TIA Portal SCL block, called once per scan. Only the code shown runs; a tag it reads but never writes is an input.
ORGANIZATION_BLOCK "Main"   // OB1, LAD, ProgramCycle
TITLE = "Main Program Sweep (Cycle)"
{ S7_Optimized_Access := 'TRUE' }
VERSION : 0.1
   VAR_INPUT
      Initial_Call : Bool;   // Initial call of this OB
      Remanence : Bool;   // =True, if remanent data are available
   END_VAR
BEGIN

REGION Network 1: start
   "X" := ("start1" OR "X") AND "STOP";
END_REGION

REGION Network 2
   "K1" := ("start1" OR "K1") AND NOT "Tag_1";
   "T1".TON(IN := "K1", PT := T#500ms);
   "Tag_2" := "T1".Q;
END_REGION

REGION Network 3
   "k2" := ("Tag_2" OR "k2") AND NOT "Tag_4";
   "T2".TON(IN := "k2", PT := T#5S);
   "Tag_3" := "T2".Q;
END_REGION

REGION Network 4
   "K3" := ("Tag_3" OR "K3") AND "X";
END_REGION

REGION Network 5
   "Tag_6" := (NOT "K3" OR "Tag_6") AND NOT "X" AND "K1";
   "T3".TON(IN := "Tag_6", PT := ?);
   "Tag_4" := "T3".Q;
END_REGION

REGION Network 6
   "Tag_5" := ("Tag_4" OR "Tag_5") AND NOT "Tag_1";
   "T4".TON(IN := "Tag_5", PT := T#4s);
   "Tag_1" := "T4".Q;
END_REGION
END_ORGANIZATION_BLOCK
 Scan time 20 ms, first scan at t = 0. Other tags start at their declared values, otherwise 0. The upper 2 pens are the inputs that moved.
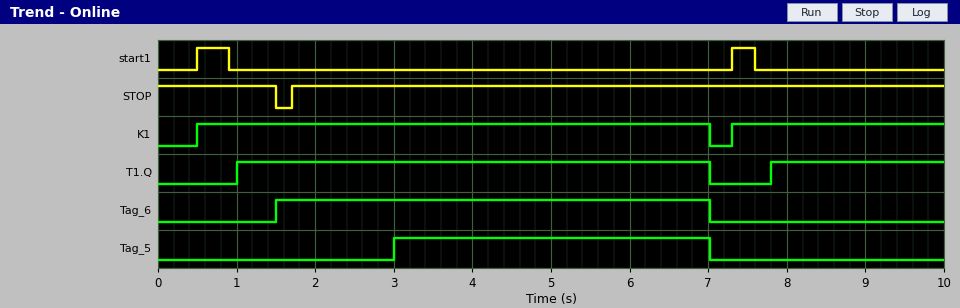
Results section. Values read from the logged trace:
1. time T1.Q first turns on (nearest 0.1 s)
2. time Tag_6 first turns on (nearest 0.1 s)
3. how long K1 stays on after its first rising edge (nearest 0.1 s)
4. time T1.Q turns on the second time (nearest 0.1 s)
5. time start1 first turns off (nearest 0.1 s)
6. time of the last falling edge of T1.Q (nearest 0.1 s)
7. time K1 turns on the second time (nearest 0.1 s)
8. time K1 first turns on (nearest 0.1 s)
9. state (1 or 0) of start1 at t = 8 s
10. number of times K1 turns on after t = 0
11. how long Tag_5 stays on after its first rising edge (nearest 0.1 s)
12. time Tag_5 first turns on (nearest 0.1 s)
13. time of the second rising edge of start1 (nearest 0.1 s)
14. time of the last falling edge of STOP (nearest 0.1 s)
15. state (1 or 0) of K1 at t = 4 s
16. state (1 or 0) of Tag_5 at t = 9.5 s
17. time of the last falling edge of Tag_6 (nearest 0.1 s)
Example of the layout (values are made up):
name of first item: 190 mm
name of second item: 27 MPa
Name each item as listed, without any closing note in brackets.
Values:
time T1.Q first turns on: 1.0 s
time Tag_6 first turns on: 1.5 s
how long K1 stays on after its first rising edge: 6.5 s
time T1.Q turns on the second time: 7.8 s
time start1 first turns off: 0.9 s
time of the last falling edge of T1.Q: 7.0 s
time K1 turns on the second time: 7.3 s
time K1 first turns on: 0.5 s
state (1 or 0) of start1 at t = 8 s: 0
number of times K1 turns on after t = 0: 2
how long Tag_5 stays on after its first rising edge: 4.0 s
time Tag_5 first turns on: 3.0 s
time of the second rising edge of start1: 7.3 s
time of the last falling edge of STOP: 1.5 s
state (1 or 0) of K1 at t = 4 s: 1
state (1 or 0) of Tag_5 at t = 9.5 s: 0
time of the last falling edge of Tag_6: 7.0 s
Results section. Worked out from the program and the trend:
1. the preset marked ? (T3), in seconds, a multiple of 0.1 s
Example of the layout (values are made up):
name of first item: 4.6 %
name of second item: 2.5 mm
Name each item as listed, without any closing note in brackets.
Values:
the preset marked ? (T3), in seconds, a multiple of 0.1 s: 1.5 s
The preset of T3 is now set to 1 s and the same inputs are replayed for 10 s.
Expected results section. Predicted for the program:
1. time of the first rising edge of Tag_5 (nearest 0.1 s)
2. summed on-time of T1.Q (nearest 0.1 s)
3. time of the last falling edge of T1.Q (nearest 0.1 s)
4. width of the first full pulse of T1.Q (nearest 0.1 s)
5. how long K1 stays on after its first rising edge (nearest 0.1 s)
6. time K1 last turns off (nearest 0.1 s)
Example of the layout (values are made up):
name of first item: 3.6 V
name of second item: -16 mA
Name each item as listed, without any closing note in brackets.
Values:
time of the first rising edge of Tag_5: 2.5 s
summed on-time of T1.Q: 7.7 s
time of the last falling edge of T1.Q: 6.5 s
width of the first full pulse of T1.Q: 5.5 s
how long K1 stays on after its first rising edge: 6.0 s
time K1 last turns off: 6.5 s
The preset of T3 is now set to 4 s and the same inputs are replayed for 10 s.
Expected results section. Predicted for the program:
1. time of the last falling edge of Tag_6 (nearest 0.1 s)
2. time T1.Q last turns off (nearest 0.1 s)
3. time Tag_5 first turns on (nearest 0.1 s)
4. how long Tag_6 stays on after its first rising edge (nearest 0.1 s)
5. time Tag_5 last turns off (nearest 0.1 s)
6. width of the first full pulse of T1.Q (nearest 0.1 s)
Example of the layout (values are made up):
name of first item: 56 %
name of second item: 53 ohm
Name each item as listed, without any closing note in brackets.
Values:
time of the last falling edge of Tag_6: 7.3 s
time T1.Q last turns off: 9.5 s
time Tag_5 first turns on: 5.5 s
how long Tag_6 stays on after its first rising edge: 5.8 s
time Tag_5 last turns off: 9.5 s
width of the first full pulse of T1.Q: 8.5 s
